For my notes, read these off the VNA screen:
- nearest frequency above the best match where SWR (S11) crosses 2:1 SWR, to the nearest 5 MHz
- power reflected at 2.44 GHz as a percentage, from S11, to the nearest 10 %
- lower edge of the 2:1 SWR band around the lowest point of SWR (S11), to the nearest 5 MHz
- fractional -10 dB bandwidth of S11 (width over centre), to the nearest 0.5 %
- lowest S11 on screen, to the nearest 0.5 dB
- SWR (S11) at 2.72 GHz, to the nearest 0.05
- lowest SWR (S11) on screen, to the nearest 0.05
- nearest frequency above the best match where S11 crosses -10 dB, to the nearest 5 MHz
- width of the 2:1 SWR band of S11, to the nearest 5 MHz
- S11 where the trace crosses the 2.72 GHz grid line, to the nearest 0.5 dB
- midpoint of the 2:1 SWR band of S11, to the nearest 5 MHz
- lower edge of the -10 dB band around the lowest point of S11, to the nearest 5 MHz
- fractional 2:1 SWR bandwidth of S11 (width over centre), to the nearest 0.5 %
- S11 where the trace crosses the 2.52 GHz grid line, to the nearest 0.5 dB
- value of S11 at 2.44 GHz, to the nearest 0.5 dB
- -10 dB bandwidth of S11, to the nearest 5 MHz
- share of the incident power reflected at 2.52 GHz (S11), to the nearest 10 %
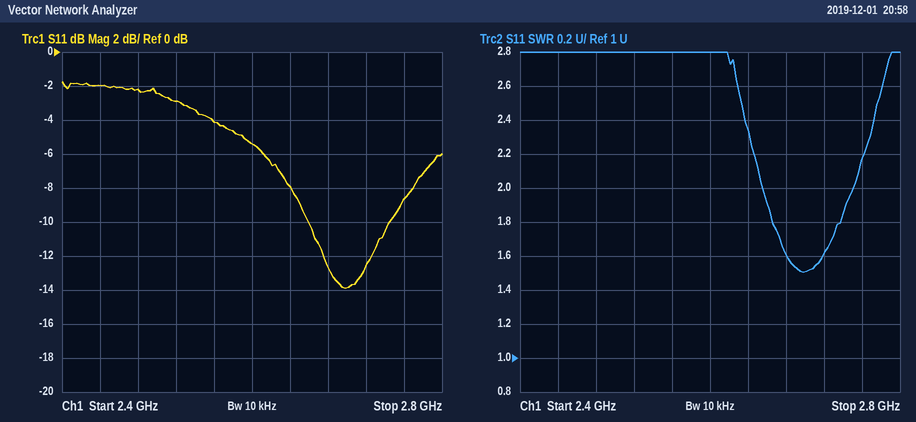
2.750 GHz
60 %
2.655 GHz
3.0 %
-14.0 dB
1.60
1.50
2.745 GHz
95 MHz
-12.5 dB
2.705 GHz
2.660 GHz
3.5 %
-3.0 dB
-2.0 dB
85 MHz
50 %
